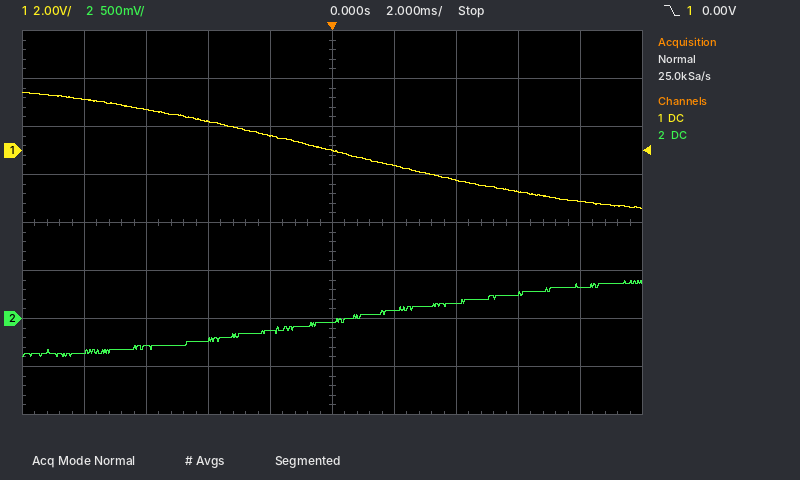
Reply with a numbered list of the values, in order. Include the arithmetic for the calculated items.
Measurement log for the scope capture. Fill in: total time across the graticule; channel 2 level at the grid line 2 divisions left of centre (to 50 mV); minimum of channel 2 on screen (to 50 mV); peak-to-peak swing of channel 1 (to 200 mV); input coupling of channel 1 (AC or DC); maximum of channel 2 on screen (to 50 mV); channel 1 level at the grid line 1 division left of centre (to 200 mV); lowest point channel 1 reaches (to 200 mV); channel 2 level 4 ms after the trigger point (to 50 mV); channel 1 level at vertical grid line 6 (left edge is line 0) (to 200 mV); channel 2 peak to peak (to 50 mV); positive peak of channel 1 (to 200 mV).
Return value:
1. 20 ms
2. -200 mV
3. -400 mV
4. 2.4 V − (-2.4 V) = 4.8 V
5. DC
6. 400 mV
7. 600 mV
8. -2.4 V
9. 150 mV
10. -600 mV
11. 400 mV − (-400 mV) = 800 mV
12. 2.4 V
